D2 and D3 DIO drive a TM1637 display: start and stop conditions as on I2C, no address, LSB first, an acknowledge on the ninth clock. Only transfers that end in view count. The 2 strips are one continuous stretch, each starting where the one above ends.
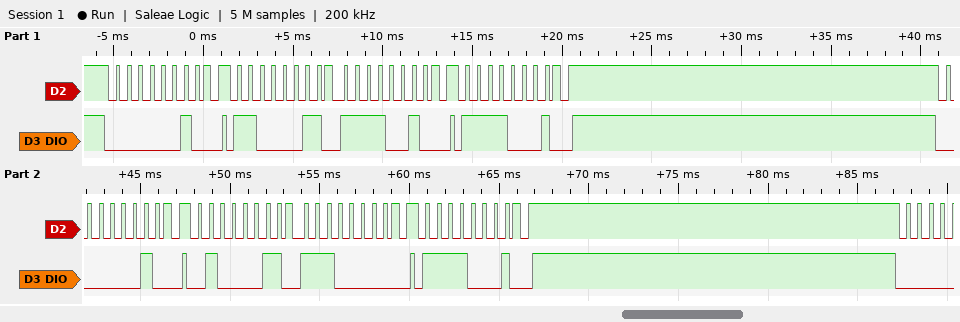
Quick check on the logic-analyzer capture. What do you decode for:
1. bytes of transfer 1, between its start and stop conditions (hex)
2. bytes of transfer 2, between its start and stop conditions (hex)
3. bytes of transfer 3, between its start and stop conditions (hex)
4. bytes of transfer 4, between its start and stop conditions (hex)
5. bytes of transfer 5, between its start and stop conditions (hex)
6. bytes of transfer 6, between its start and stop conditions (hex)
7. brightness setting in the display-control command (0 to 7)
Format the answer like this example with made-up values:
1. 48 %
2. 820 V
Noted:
1. 40
2. C3 4F
3. 8F
4. 40
5. C2 07
6. 8F
7. 7
